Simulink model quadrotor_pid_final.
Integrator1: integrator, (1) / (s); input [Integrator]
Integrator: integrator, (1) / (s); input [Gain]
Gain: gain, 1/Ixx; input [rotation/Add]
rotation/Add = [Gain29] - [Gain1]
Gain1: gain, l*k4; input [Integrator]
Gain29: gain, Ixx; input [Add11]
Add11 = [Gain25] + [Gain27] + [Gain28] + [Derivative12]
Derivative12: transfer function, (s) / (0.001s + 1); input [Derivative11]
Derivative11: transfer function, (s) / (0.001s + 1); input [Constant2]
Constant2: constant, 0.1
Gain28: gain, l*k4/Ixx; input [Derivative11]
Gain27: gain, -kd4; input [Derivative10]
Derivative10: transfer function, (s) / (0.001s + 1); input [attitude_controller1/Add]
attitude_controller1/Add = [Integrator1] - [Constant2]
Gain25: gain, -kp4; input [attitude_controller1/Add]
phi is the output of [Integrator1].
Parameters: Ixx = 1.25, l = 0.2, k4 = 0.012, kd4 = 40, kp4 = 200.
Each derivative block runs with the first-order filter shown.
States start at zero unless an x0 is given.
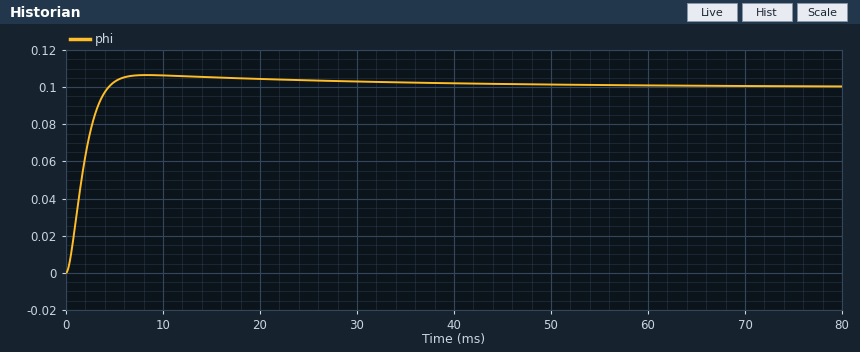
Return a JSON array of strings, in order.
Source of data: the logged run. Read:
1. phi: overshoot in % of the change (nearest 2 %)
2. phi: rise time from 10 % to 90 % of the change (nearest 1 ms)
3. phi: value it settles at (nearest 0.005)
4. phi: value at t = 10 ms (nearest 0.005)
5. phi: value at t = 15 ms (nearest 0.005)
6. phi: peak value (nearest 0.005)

["6 %", "3 ms", "0.100", "0.105", "0.105", "0.105"]
